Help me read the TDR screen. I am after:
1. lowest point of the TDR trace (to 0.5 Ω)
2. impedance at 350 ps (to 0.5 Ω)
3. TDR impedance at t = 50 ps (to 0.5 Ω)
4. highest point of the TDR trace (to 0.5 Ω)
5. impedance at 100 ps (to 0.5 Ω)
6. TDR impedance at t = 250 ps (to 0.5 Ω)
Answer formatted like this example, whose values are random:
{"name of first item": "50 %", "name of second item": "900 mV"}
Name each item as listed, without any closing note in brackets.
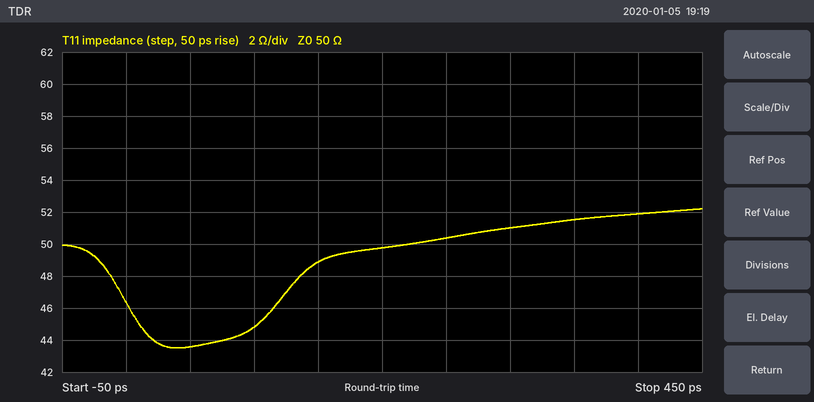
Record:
{"lowest point of the TDR trace": "43.5 Ω", "impedance at 350 ps": "51.5 Ω", "TDR impedance at t = 50 ps": "43.5 Ω", "highest point of the TDR trace": "52.0 Ω", "impedance at 100 ps": "45.0 Ω", "TDR impedance at t = 250 ps": "50.5 Ω"}
